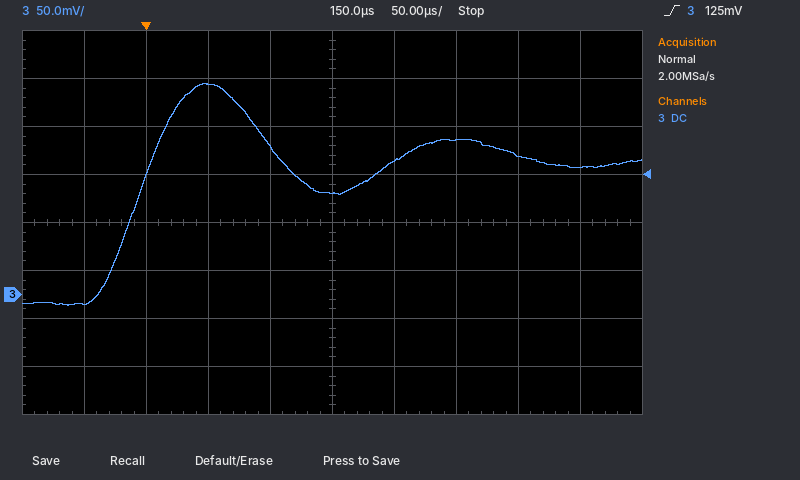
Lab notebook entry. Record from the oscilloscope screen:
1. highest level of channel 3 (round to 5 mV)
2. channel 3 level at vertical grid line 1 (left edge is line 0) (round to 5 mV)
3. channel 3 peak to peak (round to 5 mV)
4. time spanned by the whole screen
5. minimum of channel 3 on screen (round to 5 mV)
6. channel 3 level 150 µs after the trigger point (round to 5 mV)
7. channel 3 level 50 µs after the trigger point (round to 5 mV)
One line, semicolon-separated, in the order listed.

220 mV; -10 mV; 230 mV; 500 µs; -10 mV; 105 mV; 220 mV
